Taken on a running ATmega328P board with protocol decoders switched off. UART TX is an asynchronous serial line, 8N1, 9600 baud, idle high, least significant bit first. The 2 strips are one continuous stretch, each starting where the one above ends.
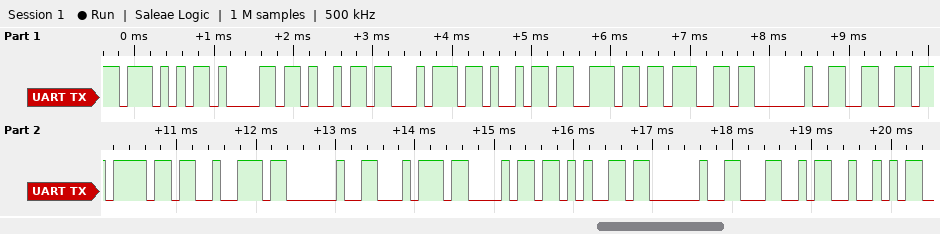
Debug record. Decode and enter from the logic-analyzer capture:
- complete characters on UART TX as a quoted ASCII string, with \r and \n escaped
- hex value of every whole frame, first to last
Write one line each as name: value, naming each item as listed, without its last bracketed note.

complete characters on UART TX as a quoted ASCII string, with \r and \n escaped: "Waiting for the LR"
hex value of every whole frame, first to last: 57 61 69 74 69 6E 67 20 66 6F 72 20 74 68 65 20 4C 52
